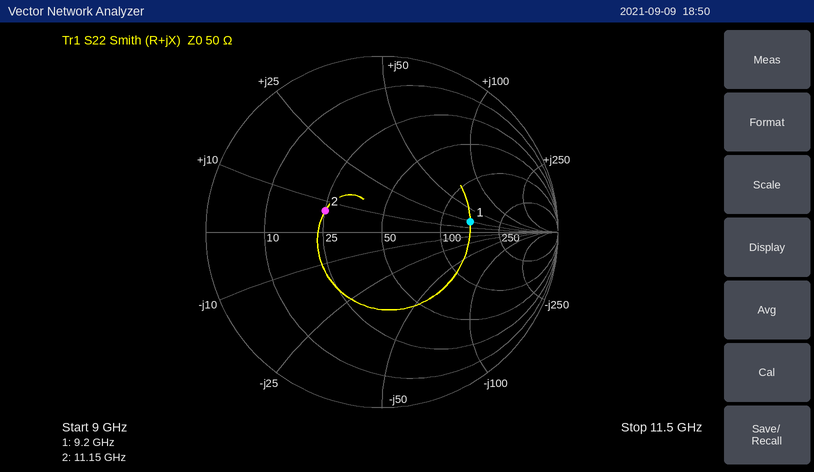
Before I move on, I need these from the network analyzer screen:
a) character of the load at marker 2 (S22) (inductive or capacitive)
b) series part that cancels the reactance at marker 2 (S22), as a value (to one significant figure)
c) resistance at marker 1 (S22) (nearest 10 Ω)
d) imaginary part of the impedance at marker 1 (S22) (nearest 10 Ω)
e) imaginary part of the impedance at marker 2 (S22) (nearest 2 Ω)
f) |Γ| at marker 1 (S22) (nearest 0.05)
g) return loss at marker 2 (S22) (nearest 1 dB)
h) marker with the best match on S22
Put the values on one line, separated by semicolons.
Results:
inductive; 2 pF; 150 Ω; +20 Ω; +6 Ω; 0.50; 9 dB; marker 2
